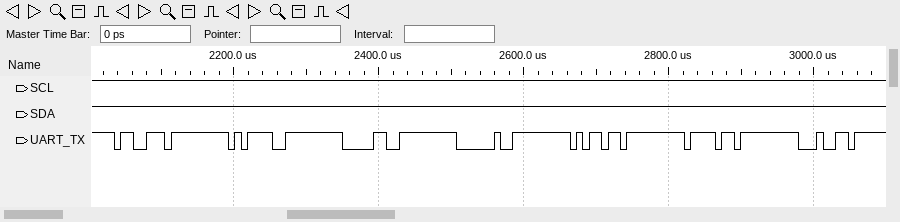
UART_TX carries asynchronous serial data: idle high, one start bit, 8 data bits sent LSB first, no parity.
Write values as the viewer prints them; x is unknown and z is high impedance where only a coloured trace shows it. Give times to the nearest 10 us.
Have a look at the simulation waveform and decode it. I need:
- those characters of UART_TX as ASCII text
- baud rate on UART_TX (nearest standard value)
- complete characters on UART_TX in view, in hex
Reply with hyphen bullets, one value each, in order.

- "s=0 mod"
- 115200 baud
- 73, 3D, 30, 20, 6D, 6F, 64
